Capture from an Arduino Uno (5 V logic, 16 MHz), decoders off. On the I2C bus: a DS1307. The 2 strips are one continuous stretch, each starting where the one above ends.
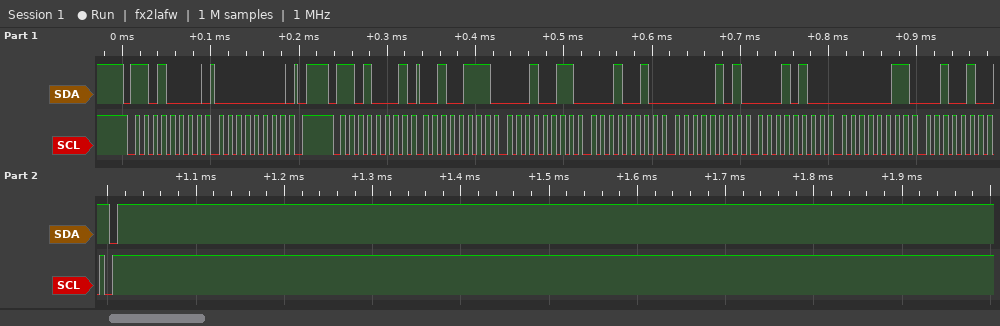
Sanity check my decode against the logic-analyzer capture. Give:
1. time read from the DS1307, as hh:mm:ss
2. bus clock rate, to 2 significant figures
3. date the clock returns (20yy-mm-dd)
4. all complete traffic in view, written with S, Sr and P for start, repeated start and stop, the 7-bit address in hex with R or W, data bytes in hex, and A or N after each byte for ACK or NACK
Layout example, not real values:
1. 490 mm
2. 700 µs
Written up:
1. 12:13:27
2. 100 kHz
3. 2024-03-14
4. S 68W A 00 A P S 68R A 27 A 13 A 12 A 05 A 14 A 03 A 24 N P
